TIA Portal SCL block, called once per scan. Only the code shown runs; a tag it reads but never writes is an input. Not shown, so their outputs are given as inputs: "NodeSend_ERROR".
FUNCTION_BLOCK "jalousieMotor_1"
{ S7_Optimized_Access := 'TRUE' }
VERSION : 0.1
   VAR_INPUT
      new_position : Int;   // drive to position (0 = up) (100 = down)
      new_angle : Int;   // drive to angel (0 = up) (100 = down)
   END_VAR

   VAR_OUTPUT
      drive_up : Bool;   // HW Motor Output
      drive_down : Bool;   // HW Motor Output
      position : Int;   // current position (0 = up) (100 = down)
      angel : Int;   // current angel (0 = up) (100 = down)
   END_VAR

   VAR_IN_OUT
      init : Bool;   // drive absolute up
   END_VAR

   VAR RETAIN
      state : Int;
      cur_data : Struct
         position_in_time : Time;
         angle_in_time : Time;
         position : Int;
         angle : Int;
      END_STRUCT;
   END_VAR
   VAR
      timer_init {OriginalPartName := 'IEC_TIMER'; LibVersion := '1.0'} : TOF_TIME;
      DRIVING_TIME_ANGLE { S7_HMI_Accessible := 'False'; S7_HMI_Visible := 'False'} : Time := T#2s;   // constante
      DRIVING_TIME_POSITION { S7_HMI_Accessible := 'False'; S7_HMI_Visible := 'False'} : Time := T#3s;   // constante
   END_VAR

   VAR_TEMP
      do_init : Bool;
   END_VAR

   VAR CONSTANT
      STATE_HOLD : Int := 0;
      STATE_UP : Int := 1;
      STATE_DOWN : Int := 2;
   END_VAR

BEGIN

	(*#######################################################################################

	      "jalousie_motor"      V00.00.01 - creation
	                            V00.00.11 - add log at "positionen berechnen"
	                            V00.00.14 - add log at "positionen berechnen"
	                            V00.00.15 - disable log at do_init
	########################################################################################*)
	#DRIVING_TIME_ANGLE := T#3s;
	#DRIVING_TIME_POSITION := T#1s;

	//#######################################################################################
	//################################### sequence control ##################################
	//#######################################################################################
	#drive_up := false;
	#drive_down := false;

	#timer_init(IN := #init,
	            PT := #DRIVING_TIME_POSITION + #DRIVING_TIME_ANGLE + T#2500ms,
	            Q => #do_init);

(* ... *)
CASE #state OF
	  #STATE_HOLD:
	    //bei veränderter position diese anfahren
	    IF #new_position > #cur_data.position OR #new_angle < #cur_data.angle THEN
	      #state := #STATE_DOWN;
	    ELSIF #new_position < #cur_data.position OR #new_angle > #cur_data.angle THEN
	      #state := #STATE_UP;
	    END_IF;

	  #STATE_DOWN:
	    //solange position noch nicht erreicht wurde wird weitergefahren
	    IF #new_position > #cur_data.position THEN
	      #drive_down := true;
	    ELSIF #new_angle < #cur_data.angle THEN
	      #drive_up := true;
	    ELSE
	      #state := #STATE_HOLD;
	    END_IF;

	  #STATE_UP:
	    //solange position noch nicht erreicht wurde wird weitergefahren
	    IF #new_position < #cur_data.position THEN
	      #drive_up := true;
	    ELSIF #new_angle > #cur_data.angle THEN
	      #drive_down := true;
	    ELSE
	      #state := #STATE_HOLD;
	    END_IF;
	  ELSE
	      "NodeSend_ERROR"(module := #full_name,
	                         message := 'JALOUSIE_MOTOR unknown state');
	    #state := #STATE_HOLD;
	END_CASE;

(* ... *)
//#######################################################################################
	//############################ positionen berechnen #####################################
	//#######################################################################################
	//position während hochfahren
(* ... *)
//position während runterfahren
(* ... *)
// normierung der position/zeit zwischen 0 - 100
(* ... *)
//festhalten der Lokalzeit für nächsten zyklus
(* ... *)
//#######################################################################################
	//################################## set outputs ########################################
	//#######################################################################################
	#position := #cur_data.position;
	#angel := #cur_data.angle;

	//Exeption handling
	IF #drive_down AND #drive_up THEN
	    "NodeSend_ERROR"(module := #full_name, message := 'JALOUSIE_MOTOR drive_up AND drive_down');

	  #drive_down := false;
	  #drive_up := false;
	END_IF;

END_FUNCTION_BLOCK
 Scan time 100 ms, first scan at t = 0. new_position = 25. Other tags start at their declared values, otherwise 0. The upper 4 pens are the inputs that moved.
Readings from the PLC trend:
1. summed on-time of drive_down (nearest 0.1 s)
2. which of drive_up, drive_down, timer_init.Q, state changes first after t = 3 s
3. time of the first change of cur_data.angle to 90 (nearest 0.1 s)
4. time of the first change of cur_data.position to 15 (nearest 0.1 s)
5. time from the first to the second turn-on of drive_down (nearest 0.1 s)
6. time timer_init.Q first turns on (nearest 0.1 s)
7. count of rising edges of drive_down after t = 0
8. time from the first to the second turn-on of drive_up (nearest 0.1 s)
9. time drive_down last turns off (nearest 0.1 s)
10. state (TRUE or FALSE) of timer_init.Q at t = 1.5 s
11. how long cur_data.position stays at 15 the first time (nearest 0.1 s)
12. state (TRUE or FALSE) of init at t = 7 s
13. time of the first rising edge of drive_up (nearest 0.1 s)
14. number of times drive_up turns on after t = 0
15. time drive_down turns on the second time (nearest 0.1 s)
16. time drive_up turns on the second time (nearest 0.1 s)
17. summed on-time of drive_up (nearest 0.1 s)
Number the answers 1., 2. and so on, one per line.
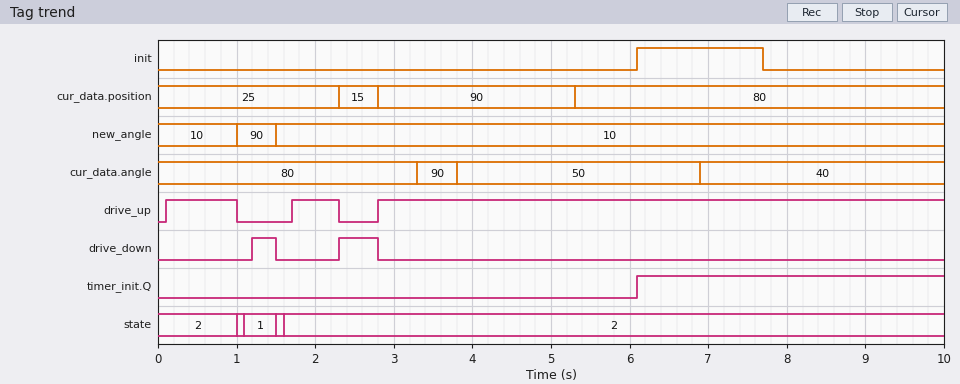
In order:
1. 0.8 s
2. timer_init.Q
3. 3.3 s
4. 2.3 s
5. 1.1 s
6. 6.1 s
7. 2
8. 1.6 s
9. 2.8 s
10. FALSE
11. 0.5 s
12. TRUE
13. 0.1 s
14. 3
15. 2.3 s
16. 1.7 s
17. 8.7 s
